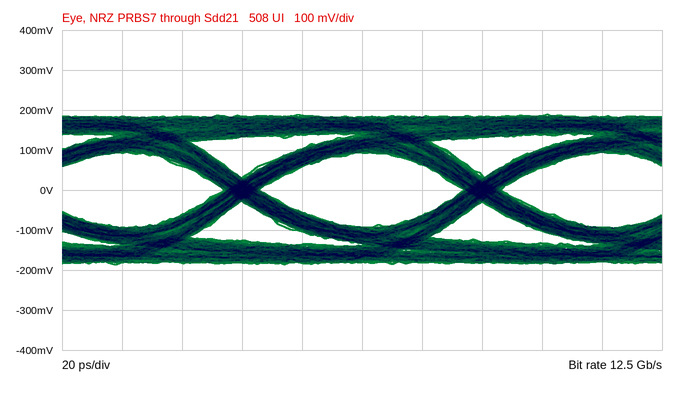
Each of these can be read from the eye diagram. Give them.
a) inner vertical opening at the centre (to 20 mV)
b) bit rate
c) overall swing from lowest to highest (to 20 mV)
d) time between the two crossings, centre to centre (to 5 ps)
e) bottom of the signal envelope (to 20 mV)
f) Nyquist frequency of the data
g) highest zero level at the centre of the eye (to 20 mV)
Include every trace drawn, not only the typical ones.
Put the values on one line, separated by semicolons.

180 mV; 12.5 Gb/s; 380 mV; 80 ps; -180 mV; 6.25 GHz; -100 mV
